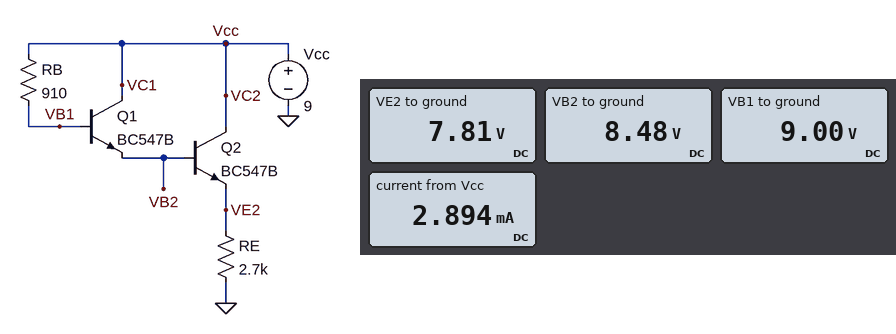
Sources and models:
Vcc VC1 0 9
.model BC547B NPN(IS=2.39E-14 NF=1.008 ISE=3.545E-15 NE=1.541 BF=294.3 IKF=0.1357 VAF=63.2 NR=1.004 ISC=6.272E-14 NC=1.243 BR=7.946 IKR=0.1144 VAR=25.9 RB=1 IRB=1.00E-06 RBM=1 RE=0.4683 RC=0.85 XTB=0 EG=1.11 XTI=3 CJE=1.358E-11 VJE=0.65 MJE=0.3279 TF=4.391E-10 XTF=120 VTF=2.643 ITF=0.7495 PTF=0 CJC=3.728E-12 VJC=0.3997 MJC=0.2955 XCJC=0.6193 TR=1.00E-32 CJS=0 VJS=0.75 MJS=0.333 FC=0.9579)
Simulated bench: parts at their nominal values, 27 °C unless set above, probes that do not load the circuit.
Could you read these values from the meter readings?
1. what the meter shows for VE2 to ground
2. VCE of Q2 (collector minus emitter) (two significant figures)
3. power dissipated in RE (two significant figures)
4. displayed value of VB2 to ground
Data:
7.81 V
1.2 V
23 mW
8.48 V
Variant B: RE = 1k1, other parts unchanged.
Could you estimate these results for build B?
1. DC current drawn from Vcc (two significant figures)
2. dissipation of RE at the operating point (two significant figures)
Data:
7.1 mA
55 mW
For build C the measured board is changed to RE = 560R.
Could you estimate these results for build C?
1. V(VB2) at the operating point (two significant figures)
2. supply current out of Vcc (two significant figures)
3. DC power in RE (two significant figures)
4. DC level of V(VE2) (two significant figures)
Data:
8.4 V
14 mA
110 mW
7.7 V
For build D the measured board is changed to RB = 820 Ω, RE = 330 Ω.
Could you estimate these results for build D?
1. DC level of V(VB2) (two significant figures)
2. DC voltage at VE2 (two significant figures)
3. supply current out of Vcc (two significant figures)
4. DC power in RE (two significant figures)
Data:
8.4 V
7.7 V
23 mA
180 mW
